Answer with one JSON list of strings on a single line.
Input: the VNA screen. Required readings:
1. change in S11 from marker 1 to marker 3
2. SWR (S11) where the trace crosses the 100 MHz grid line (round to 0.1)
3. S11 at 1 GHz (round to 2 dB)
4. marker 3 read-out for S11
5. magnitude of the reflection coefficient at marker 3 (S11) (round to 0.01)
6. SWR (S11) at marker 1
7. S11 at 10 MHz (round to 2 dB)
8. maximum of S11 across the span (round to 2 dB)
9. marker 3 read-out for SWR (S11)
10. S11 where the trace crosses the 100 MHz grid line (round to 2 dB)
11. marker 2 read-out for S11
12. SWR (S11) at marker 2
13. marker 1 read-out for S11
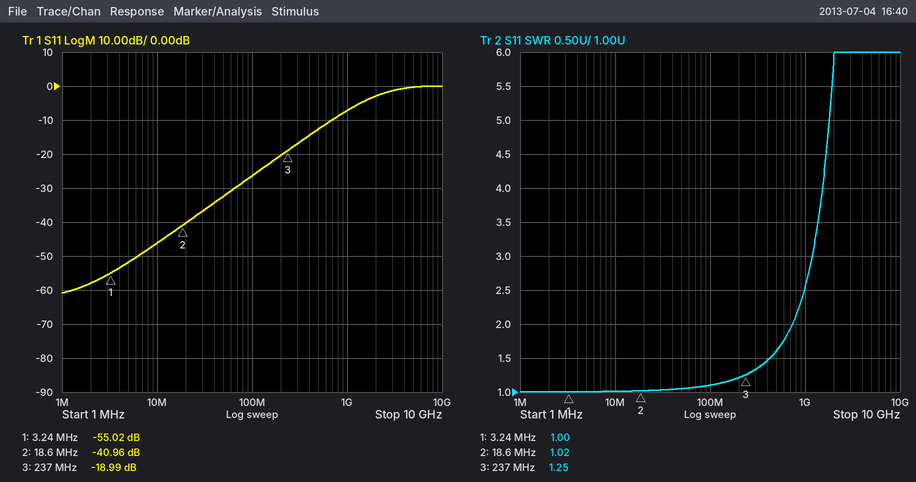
["36.03 dB", "1.1", "-8 dB", "-18.99 dB", "0.11", "1.00", "-46 dB", "0 dB", "1.25", "-26 dB", "-40.96 dB", "1.02", "-55.02 dB"]
